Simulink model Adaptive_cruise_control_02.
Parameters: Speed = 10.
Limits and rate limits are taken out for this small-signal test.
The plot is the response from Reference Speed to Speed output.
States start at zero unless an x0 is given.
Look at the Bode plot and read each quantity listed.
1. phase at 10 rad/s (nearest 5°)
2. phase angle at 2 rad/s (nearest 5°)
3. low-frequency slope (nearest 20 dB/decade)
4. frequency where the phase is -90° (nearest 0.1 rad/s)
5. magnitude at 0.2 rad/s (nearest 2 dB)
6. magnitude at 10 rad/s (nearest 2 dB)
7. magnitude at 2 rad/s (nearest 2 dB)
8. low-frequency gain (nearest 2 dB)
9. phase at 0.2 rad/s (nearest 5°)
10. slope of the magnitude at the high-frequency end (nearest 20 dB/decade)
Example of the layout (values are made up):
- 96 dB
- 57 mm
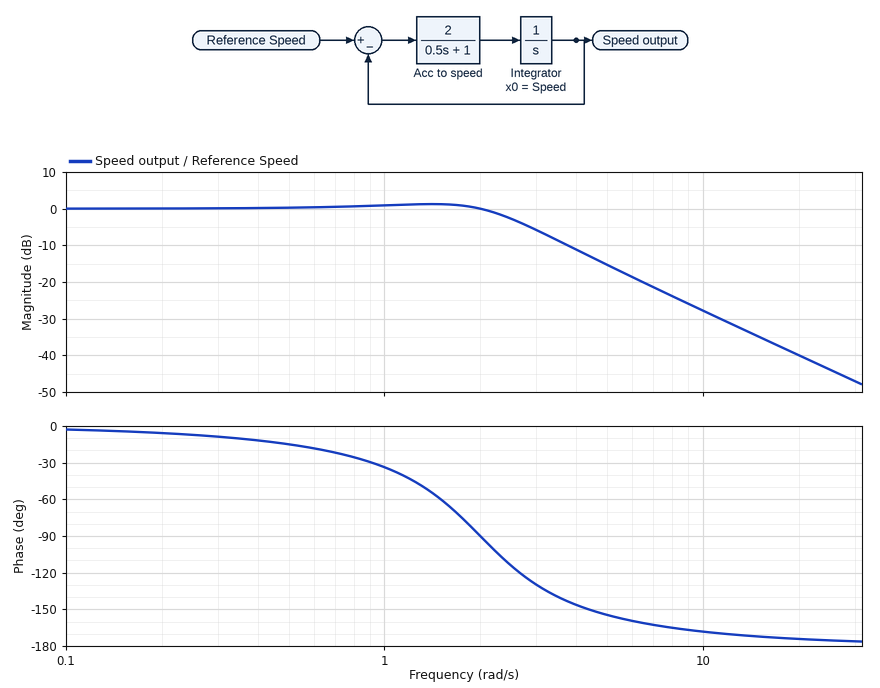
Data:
- -170°
- -90°
- 0 dB/decade
- 2.0 rad/s
- 0 dB
- -28 dB
- 0 dB
- 0 dB
- -5°
- -40 dB/decade
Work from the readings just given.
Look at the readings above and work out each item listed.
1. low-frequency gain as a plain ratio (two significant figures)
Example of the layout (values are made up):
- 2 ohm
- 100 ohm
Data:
- 1.0
